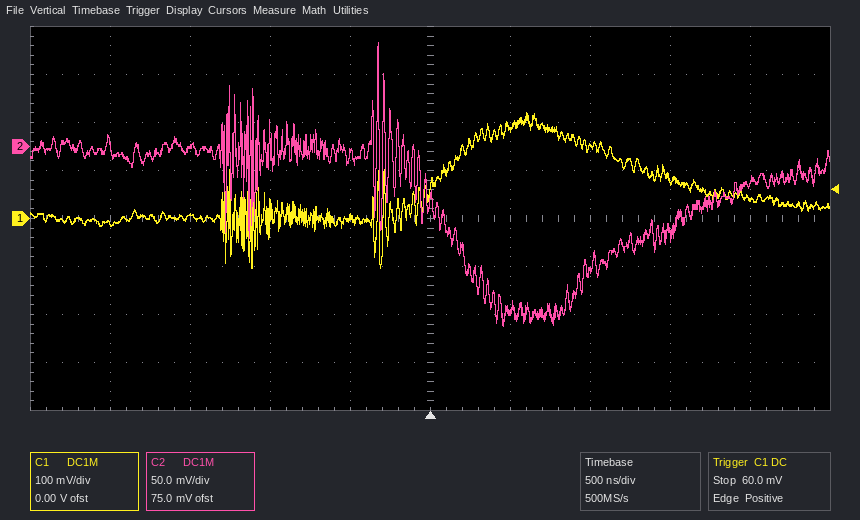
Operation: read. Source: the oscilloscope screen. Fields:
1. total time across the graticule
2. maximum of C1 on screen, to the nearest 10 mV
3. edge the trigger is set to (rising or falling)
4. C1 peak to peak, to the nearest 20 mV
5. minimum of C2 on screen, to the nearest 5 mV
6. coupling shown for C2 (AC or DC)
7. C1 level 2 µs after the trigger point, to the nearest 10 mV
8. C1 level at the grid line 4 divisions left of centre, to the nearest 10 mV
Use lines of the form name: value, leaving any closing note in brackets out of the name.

total time across the graticule: 5 µs
maximum of C1 on screen, to the nearest 10 mV: 220 mV
edge the trigger is set to: rising
C1 peak to peak, to the nearest 20 mV: 320 mV
minimum of C2 on screen, to the nearest 5 mV: -190 mV
coupling shown for C2: DC
C1 level 2 µs after the trigger point, to the nearest 10 mV: 40 mV
C1 level at the grid line 4 divisions left of centre, to the nearest 10 mV: -10 mV
